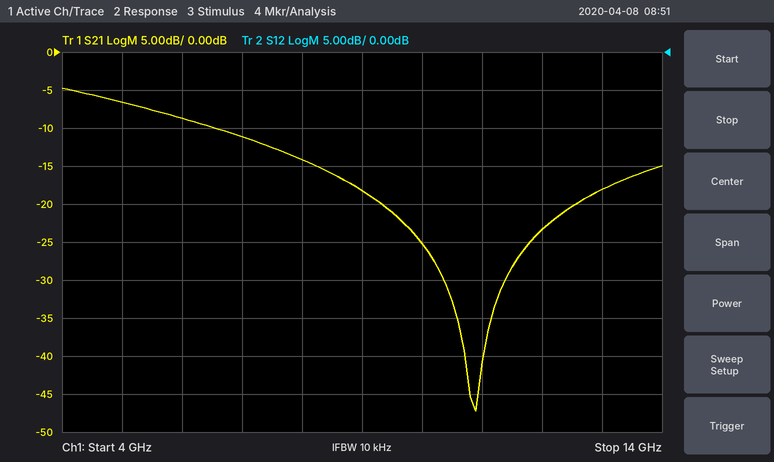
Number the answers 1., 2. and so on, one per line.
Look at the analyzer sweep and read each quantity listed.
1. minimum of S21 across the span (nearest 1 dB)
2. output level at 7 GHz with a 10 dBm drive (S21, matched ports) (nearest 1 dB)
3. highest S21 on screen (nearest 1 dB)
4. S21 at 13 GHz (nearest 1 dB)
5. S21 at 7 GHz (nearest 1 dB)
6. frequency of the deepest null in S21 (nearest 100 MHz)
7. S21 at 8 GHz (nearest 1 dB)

1. -47 dB
2. -1 dBm
3. -5 dB
4. -18 dB
5. -11 dB
6. 10.9 GHz
7. -14 dB
